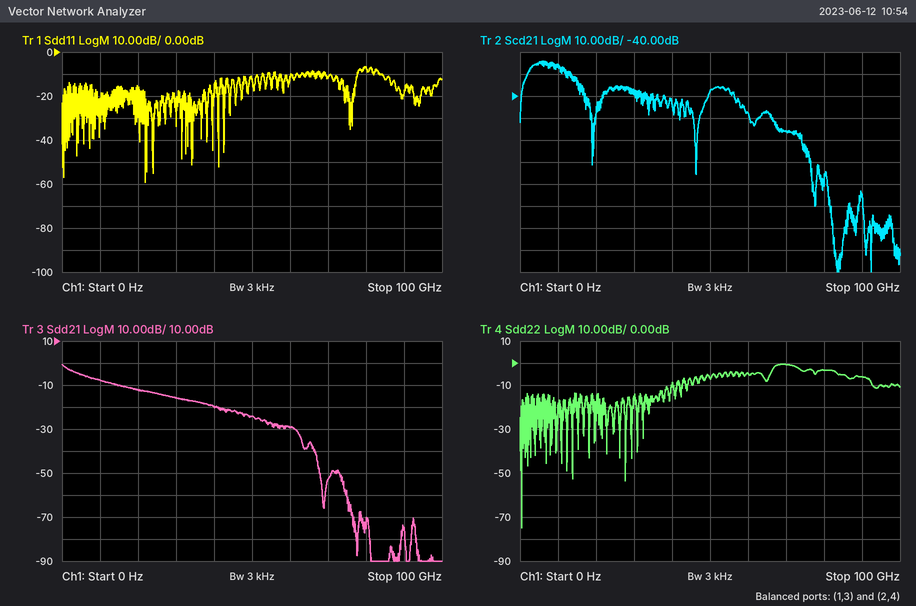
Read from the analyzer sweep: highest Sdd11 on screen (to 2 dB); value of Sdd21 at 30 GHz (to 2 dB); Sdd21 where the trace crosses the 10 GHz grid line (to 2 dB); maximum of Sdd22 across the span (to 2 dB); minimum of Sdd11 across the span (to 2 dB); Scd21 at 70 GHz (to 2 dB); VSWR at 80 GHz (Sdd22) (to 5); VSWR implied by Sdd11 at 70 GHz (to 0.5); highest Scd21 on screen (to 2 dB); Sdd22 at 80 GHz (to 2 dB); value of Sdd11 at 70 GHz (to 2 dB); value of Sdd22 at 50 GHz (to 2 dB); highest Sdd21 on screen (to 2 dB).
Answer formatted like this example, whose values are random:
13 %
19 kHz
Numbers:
-6 dB
-16 dB
-8 dB
0 dB
-60 dB
-56 dB
5
1.5
-24 dB
-4 dB
-12 dB
-6 dB
0 dB
